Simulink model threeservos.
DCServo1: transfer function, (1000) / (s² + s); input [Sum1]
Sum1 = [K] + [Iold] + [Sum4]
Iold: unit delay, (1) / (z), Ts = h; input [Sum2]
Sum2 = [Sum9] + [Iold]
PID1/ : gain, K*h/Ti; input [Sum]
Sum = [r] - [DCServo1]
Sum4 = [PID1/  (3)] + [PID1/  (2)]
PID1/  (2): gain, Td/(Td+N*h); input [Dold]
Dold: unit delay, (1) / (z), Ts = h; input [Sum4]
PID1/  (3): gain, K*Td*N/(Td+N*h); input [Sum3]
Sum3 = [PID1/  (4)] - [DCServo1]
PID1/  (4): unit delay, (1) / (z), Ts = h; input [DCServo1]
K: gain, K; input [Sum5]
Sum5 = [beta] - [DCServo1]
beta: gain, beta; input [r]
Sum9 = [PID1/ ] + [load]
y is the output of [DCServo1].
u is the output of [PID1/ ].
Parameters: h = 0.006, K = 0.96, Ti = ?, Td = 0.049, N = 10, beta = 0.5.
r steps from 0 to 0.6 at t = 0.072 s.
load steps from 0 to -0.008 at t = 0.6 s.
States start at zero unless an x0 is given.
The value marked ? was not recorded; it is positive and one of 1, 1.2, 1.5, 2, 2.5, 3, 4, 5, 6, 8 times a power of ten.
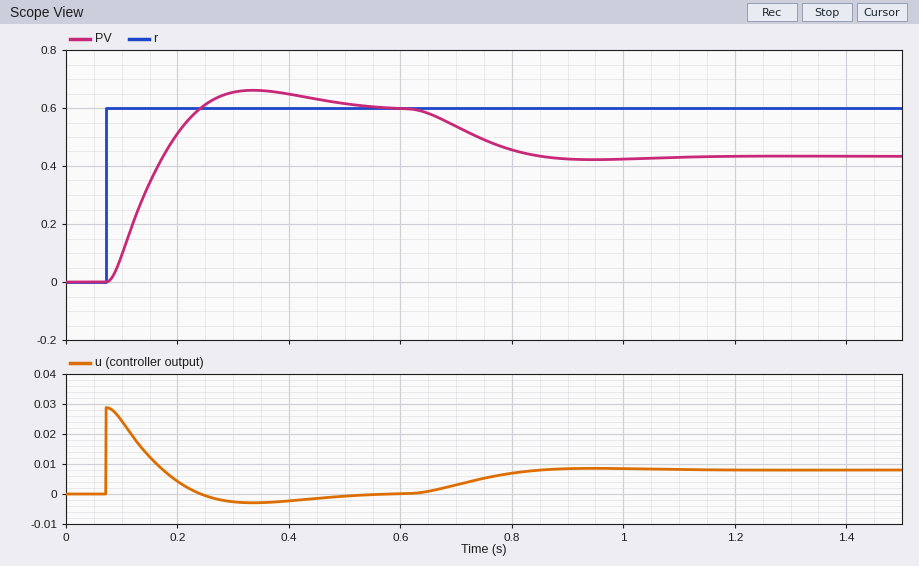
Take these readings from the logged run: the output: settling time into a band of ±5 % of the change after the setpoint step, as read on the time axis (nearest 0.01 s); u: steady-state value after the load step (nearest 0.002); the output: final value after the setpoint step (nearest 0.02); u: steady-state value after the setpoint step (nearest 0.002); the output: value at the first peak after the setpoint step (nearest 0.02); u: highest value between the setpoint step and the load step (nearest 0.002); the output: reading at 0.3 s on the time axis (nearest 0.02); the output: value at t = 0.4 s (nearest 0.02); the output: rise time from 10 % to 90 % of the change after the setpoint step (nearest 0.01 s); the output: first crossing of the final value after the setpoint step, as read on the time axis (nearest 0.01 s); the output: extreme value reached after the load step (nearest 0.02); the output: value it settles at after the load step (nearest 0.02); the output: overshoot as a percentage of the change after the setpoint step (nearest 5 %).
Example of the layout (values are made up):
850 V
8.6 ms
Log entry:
0.45 s
0.008
0.60
0.000
0.66
0.028
0.66
0.64
0.12 s
0.24 s
0.42
0.44
10 %
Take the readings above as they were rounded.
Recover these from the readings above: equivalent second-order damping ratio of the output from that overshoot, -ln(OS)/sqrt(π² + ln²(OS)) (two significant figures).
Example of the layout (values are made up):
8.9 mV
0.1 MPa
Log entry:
0.59
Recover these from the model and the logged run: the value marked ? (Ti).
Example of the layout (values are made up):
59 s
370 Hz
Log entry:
0.12
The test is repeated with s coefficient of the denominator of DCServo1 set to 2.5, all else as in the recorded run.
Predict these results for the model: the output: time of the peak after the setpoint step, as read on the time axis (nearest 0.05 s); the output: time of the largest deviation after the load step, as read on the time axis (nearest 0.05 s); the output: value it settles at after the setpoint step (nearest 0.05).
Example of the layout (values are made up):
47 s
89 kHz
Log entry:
0.35 s
0.95 s
0.60
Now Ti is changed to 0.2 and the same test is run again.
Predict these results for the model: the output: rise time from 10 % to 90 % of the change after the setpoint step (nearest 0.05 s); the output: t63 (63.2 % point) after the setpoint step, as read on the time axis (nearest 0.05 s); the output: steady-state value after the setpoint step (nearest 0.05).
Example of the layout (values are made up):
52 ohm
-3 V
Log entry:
0.20 s
0.20 s
0.60
